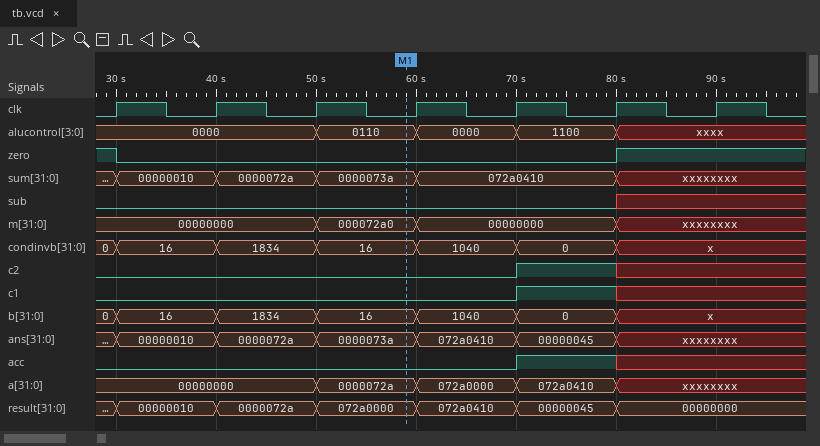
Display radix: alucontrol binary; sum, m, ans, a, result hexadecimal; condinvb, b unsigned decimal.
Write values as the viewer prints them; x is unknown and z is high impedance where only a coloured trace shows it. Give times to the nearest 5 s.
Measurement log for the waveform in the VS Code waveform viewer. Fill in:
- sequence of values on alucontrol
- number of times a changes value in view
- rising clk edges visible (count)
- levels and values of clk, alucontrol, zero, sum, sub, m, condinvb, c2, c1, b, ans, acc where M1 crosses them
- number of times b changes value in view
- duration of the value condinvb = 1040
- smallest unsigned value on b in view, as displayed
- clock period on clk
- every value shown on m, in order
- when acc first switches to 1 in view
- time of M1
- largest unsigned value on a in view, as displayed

0000, 0110, 0000, 1100, xxxx
4
7
clk=0, alucontrol=0110, zero=0, sum=0000073a, sub=0, m=000072a0, condinvb=16, c2=0, c1=0, b=16, ans=0000073a, acc=0
6
10 s
0
10 s
00000000, 000072a0, 00000000, xxxxxxxx
70 s
60 s
072a0410
